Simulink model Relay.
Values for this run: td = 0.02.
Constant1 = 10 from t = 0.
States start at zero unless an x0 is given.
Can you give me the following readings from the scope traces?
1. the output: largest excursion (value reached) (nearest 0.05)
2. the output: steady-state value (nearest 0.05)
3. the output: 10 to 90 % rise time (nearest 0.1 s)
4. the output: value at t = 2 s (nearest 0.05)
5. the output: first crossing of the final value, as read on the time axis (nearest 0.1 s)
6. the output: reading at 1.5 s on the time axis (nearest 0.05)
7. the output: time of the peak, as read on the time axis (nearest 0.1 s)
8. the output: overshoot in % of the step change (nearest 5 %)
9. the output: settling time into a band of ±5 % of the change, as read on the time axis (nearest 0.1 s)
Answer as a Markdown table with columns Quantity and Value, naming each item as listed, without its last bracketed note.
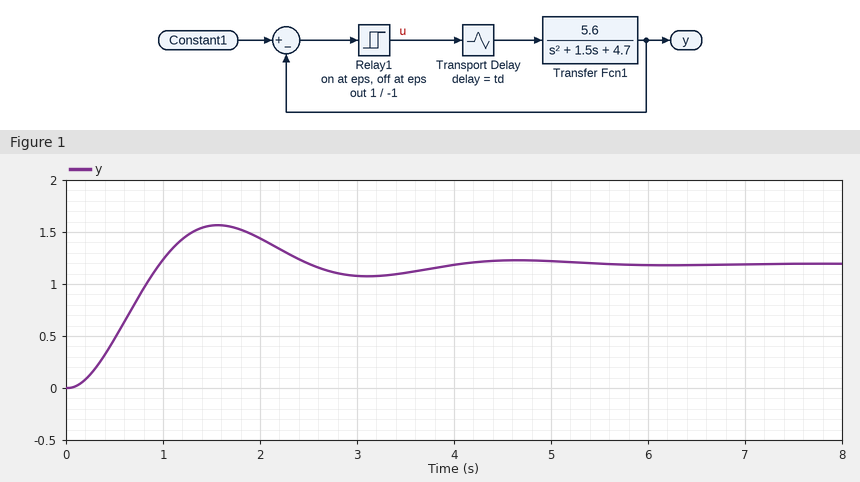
| Quantity | Value |
|---|---|
| the output: largest excursion (value reached) | 1.55 |
| the output: steady-state value | 1.20 |
| the output: 10 to 90 % rise time | 0.6 s |
| the output: value at t = 2 s | 1.45 |
| the output: first crossing of the final value, as read on the time axis | 1.0 s |
| the output: reading at 1.5 s on the time axis | 1.55 |
| the output: time of the peak, as read on the time axis | 1.6 s |
| the output: overshoot in % of the step change | 30 % |
| the output: settling time into a band of ±5 % of the change, as read on the time axis | 3.7 s |
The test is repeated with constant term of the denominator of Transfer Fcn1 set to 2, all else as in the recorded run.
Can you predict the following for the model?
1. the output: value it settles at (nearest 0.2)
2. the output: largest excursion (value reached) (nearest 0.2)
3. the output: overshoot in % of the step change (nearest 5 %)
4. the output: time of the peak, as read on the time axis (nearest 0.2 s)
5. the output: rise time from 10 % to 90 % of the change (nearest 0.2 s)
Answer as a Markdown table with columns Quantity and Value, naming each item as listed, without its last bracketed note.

| Quantity | Value |
|---|---|
| the output: value it settles at | 2.8 |
| the output: largest excursion (value reached) | 3.2 |
| the output: overshoot in % of the step change | 15 % |
| the output: time of the peak, as read on the time axis | 2.6 s |
| the output: rise time from 10 % to 90 % of the change | 1.2 s |
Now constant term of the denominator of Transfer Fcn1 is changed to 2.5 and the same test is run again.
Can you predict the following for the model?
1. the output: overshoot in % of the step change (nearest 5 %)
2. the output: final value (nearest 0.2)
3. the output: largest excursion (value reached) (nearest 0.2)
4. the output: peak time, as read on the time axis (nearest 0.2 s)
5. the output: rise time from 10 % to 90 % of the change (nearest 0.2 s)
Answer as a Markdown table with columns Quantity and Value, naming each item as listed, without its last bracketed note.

| Quantity | Value |
|---|---|
| the output: overshoot in % of the step change | 20 % |
| the output: final value | 2.2 |
| the output: largest excursion (value reached) | 2.6 |
| the output: peak time, as read on the time axis | 2.2 s |
| the output: rise time from 10 % to 90 % of the change | 1.0 s |
